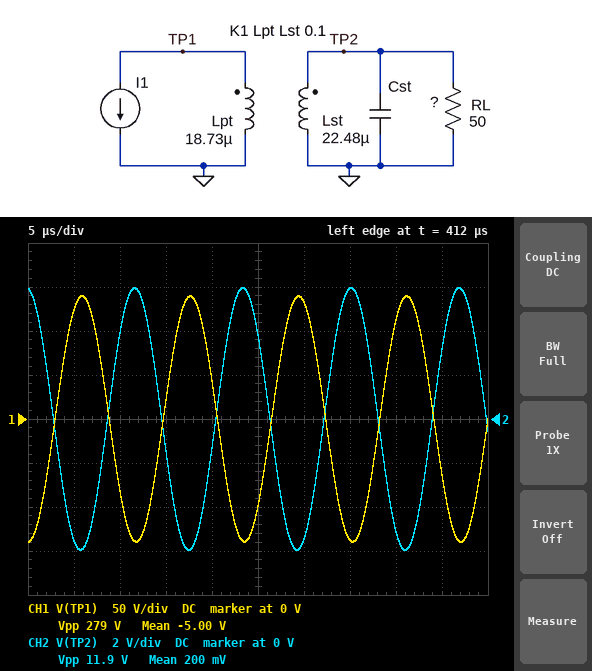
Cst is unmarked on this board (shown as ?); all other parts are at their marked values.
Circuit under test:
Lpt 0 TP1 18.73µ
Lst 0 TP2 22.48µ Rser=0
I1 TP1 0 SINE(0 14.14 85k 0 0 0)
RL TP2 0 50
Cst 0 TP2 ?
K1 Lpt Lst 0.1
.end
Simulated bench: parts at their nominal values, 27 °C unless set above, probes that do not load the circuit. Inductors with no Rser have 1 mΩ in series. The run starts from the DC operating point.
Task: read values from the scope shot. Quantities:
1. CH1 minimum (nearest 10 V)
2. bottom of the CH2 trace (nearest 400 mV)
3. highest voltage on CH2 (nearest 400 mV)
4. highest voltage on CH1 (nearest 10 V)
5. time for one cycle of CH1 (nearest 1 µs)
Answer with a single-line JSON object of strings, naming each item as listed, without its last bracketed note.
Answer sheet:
{"CH1 minimum": "-140 V", "bottom of the CH2 trace": "-6.0 V", "highest voltage on CH2": "6.0 V", "highest voltage on CH1": "140 V", "time for one cycle of CH1": "12 µs"}
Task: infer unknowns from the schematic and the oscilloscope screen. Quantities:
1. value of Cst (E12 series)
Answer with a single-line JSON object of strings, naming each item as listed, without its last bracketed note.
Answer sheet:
{"value of Cst": "560 nF"}
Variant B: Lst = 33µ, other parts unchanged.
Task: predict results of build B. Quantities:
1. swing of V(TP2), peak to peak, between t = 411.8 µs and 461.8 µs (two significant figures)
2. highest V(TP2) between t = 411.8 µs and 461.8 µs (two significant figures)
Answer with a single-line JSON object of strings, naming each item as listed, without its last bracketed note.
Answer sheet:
{"swing of V(TP2), peak to peak, between t = 411.8 µs and 461.8 µs": "8.8 V", "highest V(TP2) between t = 411.8 µs and 461.8 µs": "4.4 V"}
